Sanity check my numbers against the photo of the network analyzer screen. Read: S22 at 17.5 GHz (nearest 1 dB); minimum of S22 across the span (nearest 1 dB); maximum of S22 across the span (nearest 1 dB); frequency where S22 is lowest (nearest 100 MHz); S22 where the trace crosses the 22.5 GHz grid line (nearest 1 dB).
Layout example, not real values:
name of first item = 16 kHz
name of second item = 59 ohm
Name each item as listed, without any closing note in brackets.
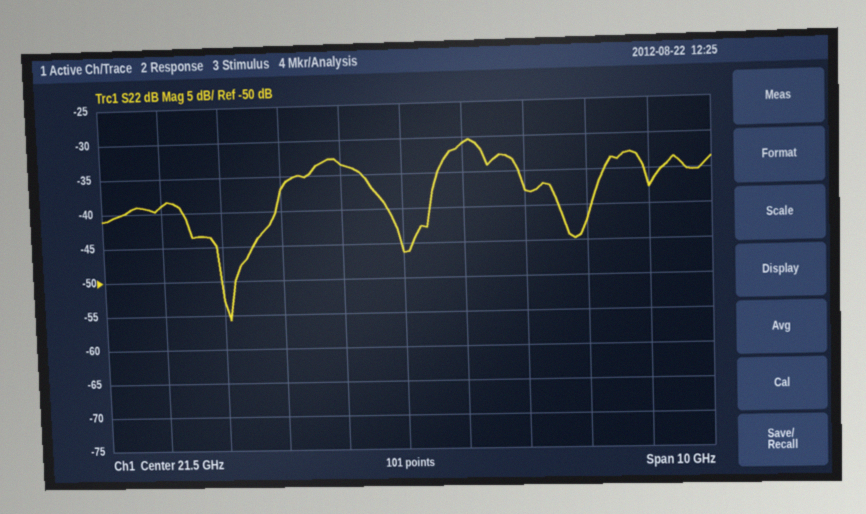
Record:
S22 at 17.5 GHz = -39 dB
minimum of S22 across the span = -56 dB
maximum of S22 across the span = -30 dB
frequency where S22 is lowest = 18.6 GHz
S22 where the trace crosses the 22.5 GHz grid line = -31 dB
